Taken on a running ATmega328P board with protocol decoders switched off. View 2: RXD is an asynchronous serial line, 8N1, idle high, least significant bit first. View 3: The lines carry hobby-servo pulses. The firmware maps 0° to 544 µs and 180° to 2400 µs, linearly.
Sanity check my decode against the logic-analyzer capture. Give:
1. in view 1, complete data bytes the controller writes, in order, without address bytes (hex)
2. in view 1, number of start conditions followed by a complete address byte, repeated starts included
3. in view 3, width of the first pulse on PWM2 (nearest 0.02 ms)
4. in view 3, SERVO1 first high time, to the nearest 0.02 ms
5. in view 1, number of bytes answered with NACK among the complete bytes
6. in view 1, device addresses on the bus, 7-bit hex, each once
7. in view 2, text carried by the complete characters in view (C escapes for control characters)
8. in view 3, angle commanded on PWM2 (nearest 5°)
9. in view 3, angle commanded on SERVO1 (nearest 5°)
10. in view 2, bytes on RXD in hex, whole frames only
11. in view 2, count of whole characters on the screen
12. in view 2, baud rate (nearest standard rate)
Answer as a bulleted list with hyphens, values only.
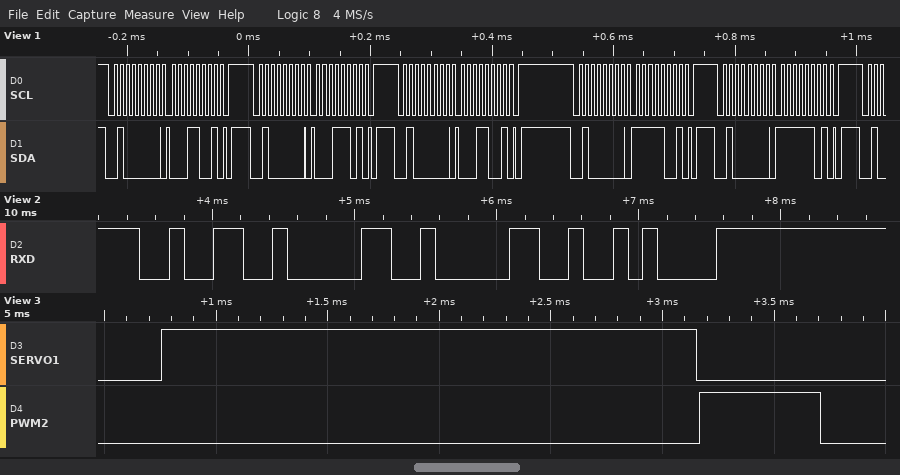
- 19 1D 19 F9 FD
- 5
- 0.54 ms
- 2.40 ms
- 0
- 0x20
- "200\n"
- 0°
- 180°
- 0x32 0x30 0x30 0x0A
- 4
- 9600 baud
